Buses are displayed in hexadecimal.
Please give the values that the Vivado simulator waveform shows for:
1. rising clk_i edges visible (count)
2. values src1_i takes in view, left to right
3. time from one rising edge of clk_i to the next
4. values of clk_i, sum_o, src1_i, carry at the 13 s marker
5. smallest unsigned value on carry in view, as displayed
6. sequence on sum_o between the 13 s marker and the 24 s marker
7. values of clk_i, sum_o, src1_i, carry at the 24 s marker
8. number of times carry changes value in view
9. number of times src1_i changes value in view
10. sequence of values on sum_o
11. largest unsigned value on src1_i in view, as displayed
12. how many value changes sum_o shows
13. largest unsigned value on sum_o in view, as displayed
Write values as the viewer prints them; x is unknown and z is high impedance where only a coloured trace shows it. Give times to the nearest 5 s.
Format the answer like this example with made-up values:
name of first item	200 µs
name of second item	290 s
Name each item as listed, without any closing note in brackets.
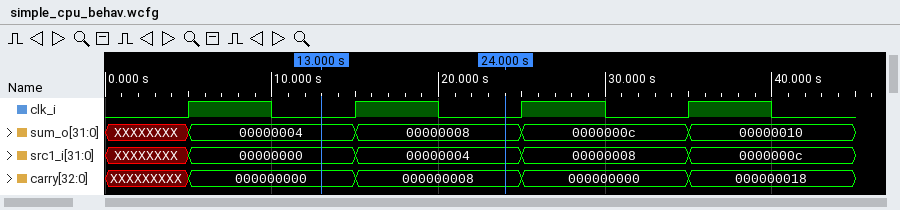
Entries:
rising clk_i edges visible	4
values src1_i takes in view, left to right	XXXXXXXX, 00000000, 00000004, 00000008, 0000000c
time from one rising edge of clk_i to the next	10 s
values of clk_i, sum_o, src1_i, carry at the 13 s marker	clk_i=0, sum_o=00000004, src1_i=00000000, carry=000000000
smallest unsigned value on carry in view, as displayed	000000000
sequence on sum_o between the 13 s marker and the 24 s marker	00000004, 00000008
values of clk_i, sum_o, src1_i, carry at the 24 s marker	clk_i=0, sum_o=00000008, src1_i=00000004, carry=000000008
number of times carry changes value in view	4
number of times src1_i changes value in view	4
sequence of values on sum_o	XXXXXXXX, 00000004, 00000008, 0000000c, 00000010
largest unsigned value on src1_i in view, as displayed	0000000c
how many value changes sum_o shows	4
largest unsigned value on sum_o in view, as displayed	00000010
